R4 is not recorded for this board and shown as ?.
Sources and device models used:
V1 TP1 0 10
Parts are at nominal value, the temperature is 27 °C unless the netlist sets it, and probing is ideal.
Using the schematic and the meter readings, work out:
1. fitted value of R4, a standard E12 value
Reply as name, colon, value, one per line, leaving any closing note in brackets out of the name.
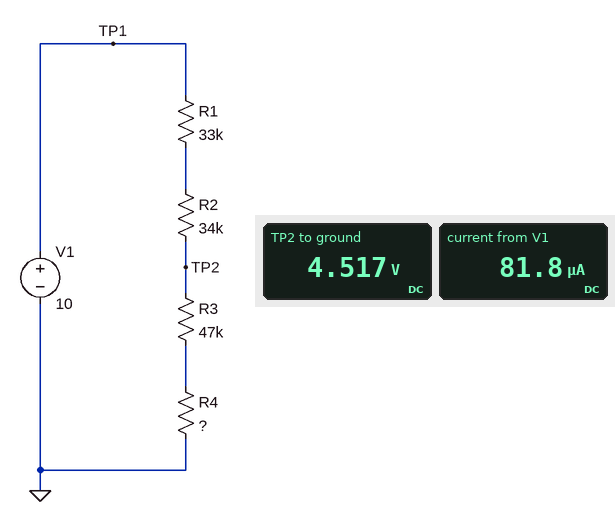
fitted value of R4, a standard E12 value: 8.2 kΩ
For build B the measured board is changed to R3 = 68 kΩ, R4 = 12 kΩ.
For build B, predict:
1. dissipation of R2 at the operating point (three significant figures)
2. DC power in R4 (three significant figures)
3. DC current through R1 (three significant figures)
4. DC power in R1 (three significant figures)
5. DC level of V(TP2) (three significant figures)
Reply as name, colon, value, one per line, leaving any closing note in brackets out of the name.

dissipation of R2 at the operating point: 157 µW
DC power in R4: 55.5 µW
DC current through R1: 68.0 µA
DC power in R1: 153 µW
DC level of V(TP2): 5.44 V
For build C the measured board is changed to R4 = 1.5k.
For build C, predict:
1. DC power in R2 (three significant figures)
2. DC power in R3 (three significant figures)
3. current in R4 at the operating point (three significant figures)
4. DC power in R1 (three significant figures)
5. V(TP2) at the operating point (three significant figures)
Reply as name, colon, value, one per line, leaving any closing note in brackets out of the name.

DC power in R2: 255 µW
DC power in R3: 352 µW
current in R4 at the operating point: 86.6 µA
DC power in R1: 247 µW
V(TP2) at the operating point: 4.20 V
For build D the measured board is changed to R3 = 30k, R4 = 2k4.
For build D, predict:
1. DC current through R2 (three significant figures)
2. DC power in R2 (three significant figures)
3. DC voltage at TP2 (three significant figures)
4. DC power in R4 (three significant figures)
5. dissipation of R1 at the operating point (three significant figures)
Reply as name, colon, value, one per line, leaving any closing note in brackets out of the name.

DC current through R2: 101 µA
DC power in R2: 344 µW
DC voltage at TP2: 3.26 V
DC power in R4: 24.3 µW
dissipation of R1 at the operating point: 334 µW
